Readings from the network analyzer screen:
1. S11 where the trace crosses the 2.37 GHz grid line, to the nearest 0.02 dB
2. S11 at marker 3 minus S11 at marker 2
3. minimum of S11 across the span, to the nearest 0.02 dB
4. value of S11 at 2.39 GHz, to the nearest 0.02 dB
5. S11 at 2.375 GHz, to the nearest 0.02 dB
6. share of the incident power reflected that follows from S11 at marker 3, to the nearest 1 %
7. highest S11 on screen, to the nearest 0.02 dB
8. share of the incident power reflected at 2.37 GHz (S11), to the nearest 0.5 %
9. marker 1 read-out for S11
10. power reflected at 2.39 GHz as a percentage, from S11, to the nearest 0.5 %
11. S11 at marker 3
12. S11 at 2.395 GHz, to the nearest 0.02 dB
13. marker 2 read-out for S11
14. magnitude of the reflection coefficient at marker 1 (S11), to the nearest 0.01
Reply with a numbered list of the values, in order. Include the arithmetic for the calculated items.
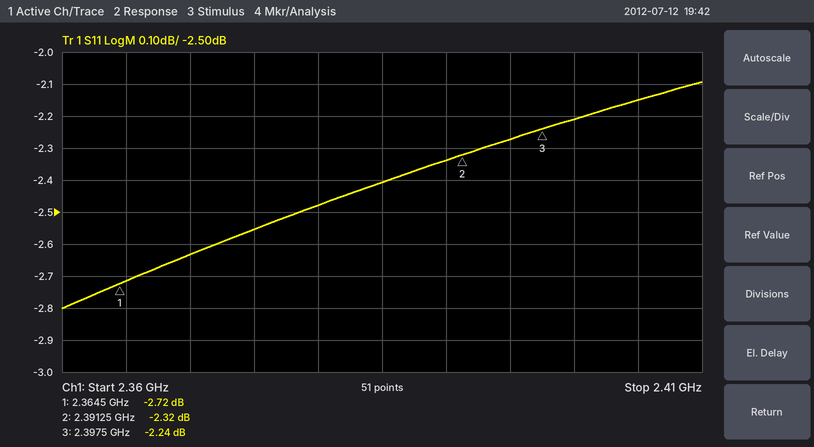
1. -2.64 dB
2. -2.24 − (-2.32) = 0.08 dB
3. -2.80 dB
4. -2.34 dB
5. -2.56 dB
6. 10^(-2.24/10) ≈ 60 %
7. -2.10 dB
8. 10^(-2.64/10) ≈ 54.5 %
9. -2.72 dB
10. 10^(-2.34/10) ≈ 58.3 %, so 58.5 % to the nearest 0.5 %
11. -2.24 dB
12. -2.28 dB
13. -2.32 dB
14. 10^(-2.72/20) ≈ 0.73
